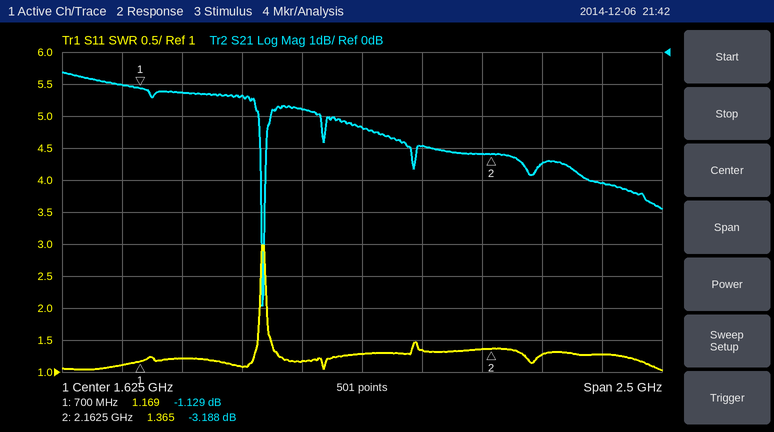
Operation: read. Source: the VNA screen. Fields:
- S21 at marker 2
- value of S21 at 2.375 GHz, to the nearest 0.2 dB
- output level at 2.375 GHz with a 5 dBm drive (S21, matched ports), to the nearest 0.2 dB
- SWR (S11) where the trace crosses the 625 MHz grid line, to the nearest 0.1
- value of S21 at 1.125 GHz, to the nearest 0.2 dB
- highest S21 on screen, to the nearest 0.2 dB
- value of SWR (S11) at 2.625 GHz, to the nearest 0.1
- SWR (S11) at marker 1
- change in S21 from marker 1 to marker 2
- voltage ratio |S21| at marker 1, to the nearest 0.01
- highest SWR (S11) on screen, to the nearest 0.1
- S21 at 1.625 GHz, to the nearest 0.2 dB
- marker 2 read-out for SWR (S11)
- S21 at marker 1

-3.188 dB
-3.4 dB
1.6 dBm
1.1
-1.4 dB
-0.6 dB
1.3
1.169
-2.059 dB
0.88
3.0
-2.4 dB
1.365
-1.129 dB
